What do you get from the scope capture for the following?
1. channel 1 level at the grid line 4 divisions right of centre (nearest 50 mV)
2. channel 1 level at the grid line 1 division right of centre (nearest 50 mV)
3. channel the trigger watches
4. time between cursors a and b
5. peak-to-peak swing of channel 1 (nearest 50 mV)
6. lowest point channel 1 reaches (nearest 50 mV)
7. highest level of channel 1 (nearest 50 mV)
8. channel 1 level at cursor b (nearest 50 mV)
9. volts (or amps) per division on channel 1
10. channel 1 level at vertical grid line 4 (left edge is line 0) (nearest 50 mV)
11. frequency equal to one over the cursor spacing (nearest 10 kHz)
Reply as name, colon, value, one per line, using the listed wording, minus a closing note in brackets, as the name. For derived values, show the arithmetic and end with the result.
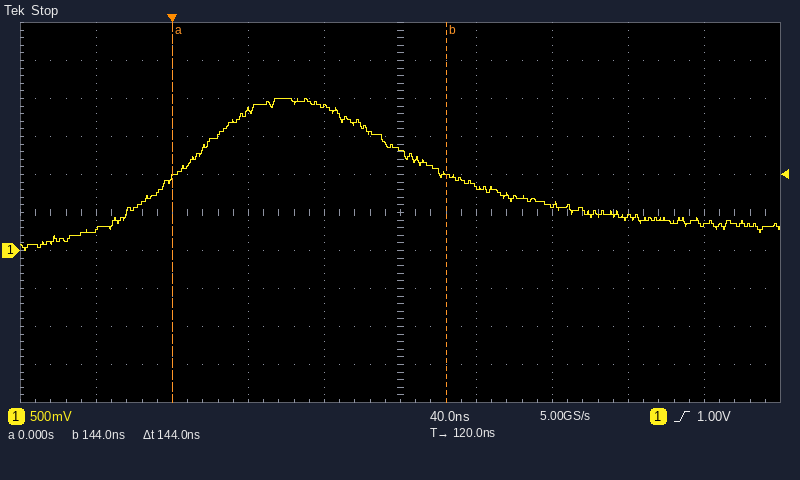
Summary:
channel 1 level at the grid line 4 divisions right of centre: 350 mV
channel 1 level at the grid line 1 division right of centre: 850 mV
channel the trigger watches: channel 1
time between cursors a and b: 144 ns
peak-to-peak swing of channel 1: 2.00 V − (0 mV) = 2.00 V
lowest point channel 1 reaches: 0 mV
highest level of channel 1: 2.00 V
channel 1 level at cursor b: 1.00 V
volts (or amps) per division on channel 1: 500 mV
channel 1 level at vertical grid line 4 (left edge is line 0): 1.90 V
frequency equal to one over the cursor spacing: 1 / 144 ns ≈ 6.94 MHz
